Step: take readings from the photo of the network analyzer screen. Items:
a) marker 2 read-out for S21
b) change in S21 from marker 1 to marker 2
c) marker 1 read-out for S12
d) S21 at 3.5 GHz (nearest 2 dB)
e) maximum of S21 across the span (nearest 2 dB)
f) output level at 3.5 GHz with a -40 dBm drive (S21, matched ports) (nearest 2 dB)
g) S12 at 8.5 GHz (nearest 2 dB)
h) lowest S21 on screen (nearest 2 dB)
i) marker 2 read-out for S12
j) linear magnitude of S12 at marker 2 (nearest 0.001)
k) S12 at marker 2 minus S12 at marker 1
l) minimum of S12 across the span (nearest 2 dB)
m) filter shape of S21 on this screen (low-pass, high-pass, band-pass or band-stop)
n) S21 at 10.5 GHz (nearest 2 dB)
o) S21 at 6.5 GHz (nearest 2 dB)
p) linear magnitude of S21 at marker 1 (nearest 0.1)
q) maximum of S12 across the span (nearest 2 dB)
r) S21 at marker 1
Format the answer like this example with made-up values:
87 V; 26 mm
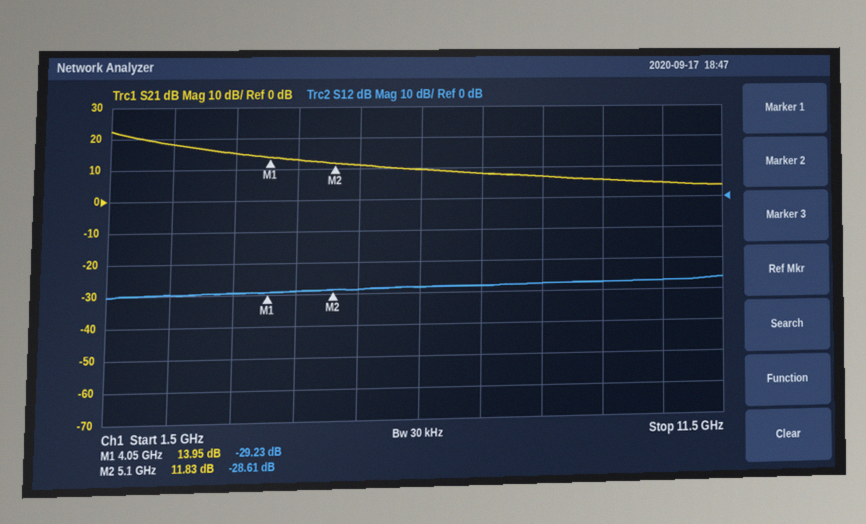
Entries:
11.83 dB; -2.12 dB; -29.23 dB; 16 dB; 22 dB; -24 dBm; -28 dB; 4 dB; -28.61 dB; 0.037; 0.62 dB; -30 dB; low-pass; 4 dB; 10 dB; 5.0; -26 dB; 13.95 dB
